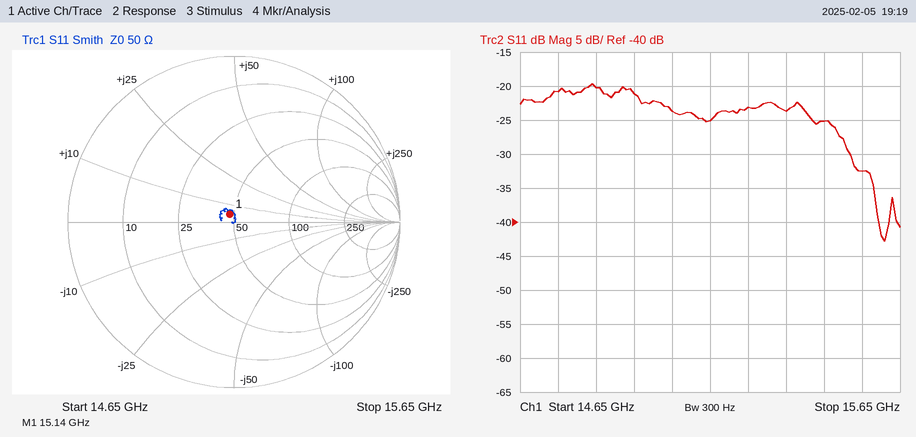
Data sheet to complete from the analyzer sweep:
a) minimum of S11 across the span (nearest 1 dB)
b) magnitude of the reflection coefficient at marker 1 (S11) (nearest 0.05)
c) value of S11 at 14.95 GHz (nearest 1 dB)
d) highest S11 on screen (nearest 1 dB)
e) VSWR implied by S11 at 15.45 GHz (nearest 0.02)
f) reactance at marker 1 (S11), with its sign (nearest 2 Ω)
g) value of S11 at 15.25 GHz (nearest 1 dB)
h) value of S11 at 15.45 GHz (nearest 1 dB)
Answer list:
-43 dB
0.05
-21 dB
-20 dB
1.12
+4 Ω
-23 dB
-25 dB
